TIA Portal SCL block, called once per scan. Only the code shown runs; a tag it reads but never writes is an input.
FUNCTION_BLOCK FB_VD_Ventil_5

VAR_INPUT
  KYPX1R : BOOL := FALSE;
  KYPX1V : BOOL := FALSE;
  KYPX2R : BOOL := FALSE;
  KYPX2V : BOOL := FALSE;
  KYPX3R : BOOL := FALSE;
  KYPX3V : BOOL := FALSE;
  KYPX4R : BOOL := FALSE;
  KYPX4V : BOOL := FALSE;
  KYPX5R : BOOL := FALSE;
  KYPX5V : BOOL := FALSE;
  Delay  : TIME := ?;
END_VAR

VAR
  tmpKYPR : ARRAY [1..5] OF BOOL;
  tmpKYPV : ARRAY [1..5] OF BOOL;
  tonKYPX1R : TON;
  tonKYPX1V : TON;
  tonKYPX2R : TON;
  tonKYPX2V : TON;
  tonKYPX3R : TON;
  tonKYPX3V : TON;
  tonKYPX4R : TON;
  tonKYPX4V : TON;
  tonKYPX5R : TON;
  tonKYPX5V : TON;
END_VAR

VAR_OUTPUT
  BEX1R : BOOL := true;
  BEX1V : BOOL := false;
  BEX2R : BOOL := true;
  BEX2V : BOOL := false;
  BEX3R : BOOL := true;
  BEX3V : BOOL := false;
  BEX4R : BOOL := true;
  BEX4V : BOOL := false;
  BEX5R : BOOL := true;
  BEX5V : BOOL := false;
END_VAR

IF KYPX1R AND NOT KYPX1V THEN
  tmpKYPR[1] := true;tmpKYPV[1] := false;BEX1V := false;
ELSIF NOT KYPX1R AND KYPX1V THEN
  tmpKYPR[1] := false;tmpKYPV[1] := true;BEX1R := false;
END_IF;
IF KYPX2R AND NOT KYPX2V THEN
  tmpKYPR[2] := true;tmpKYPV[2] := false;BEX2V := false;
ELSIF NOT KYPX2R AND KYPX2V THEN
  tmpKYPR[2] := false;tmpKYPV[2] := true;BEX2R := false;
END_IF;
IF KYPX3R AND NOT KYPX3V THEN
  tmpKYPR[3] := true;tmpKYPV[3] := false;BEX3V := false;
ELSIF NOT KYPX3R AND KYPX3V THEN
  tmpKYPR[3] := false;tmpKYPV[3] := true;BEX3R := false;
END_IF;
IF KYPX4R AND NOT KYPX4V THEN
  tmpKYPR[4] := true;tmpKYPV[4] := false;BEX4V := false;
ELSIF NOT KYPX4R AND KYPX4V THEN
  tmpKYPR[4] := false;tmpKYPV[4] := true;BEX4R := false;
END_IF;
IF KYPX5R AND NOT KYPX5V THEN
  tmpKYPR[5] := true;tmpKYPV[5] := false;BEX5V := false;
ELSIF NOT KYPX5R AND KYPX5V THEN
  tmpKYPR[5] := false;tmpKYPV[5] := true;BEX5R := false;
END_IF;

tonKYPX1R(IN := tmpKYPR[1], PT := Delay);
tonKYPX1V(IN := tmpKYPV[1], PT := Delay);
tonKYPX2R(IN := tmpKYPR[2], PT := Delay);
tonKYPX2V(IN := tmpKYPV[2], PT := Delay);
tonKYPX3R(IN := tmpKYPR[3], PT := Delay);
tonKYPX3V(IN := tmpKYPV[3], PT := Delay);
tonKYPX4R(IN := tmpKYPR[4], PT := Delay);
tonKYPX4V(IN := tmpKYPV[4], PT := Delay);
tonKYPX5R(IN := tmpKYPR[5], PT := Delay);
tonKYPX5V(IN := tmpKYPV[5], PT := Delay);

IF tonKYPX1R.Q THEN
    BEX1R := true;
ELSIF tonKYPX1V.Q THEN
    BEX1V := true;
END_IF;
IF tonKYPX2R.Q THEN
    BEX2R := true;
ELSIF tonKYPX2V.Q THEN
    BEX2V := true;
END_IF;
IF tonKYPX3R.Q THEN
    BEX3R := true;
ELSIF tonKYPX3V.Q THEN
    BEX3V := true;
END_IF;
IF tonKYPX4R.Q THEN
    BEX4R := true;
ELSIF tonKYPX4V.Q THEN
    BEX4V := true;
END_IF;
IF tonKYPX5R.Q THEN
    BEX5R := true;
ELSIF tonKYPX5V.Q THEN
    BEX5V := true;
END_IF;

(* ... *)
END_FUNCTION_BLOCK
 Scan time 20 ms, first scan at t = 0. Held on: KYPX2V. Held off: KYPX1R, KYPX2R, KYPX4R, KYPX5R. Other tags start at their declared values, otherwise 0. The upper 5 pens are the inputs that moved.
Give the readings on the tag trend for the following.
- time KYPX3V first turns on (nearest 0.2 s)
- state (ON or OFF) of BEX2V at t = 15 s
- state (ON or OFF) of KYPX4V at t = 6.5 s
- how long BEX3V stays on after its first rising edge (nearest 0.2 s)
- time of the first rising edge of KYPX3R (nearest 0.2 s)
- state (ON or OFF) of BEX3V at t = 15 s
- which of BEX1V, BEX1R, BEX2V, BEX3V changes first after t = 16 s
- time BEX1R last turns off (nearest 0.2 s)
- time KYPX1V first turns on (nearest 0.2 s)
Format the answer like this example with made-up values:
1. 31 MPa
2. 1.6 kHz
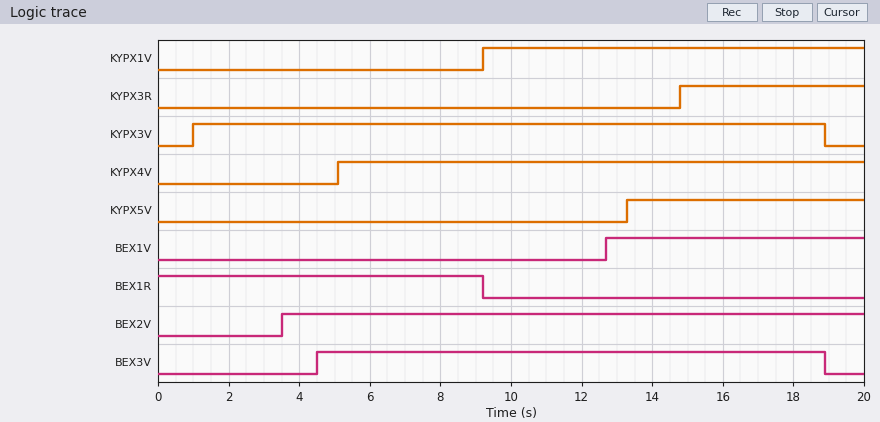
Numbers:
1. 1.0 s
2. ON
3. ON
4. 14.4 s
5. 14.8 s
6. ON
7. BEX3V
8. 9.2 s
9. 9.2 s
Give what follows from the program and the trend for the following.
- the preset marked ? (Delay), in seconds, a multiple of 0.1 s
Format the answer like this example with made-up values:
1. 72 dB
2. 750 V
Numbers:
1. 3.5 s
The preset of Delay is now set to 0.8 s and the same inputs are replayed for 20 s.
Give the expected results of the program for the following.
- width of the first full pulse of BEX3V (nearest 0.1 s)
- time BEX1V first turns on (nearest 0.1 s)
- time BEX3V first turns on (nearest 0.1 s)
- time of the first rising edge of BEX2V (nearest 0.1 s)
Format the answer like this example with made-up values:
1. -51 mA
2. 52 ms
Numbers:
1. 17.1 s
2. 10.0 s
3. 1.8 s
4. 0.8 s
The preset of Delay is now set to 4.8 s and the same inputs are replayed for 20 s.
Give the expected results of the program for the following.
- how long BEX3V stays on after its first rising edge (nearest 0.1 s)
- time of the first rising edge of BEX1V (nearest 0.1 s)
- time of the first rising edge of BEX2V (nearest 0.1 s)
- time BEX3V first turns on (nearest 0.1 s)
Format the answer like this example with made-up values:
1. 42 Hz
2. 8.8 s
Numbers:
1. 13.1 s
2. 14.0 s
3. 4.8 s
4. 5.8 s
